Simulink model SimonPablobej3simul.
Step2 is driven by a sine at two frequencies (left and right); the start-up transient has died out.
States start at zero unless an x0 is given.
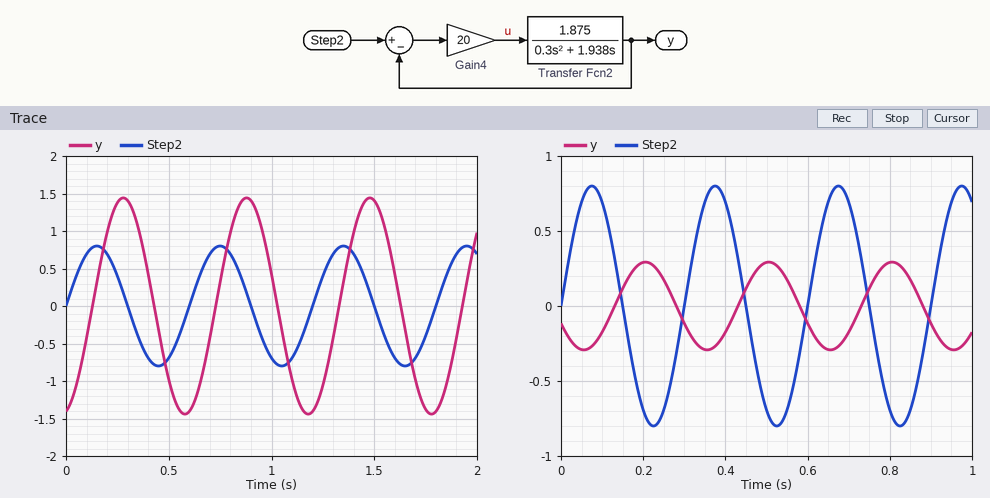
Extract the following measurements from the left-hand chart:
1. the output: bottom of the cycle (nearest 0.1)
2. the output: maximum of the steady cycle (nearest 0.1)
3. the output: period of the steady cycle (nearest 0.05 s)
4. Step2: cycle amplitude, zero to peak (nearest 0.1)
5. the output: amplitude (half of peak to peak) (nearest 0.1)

-1.4
1.4
0.60 s
0.8
1.4
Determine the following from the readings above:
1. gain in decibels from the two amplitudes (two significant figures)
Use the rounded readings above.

4.9 dB
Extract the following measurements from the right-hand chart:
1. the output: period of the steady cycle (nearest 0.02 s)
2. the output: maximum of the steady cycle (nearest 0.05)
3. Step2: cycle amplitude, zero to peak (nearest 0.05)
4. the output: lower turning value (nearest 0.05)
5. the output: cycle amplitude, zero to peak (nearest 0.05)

0.30 s
0.30
0.80
-0.30
0.30
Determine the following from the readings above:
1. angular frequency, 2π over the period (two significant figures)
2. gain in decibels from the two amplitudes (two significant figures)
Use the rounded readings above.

21 rad/s
-8.5 dB
